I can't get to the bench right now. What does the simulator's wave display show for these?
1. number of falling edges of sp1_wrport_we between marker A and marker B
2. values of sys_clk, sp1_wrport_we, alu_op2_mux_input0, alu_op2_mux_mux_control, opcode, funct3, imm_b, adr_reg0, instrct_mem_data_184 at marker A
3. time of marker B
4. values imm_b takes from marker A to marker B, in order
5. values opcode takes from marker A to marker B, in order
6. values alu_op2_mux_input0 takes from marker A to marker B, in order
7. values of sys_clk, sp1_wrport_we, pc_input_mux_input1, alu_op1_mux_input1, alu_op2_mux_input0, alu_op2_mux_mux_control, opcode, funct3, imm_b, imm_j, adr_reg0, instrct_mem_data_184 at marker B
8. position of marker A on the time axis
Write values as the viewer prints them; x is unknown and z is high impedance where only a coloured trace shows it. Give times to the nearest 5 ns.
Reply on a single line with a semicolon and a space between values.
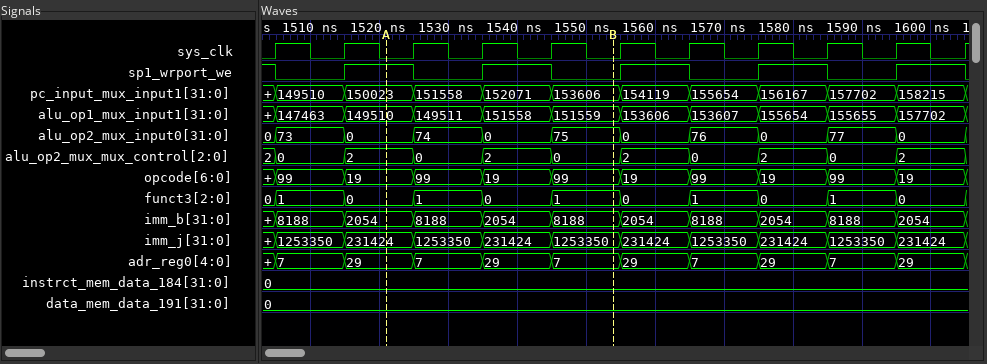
2; sys_clk=0, sp1_wrport_we=1, alu_op2_mux_input0=0, alu_op2_mux_mux_control=2, opcode=19, funct3=0, imm_b=2054, adr_reg0=29, instrct_mem_data_184=0; 1555 ns; 2054, 8188, 2054, 8188; 19, 99, 19, 99; 0, 74, 0, 75; sys_clk=0, sp1_wrport_we=0, pc_input_mux_input1=153606, alu_op1_mux_input1=151559, alu_op2_mux_input0=75, alu_op2_mux_mux_control=0, opcode=99, funct3=1, imm_b=8188, imm_j=1253350, adr_reg0=7, instrct_mem_data_184=0; 1520 ns
